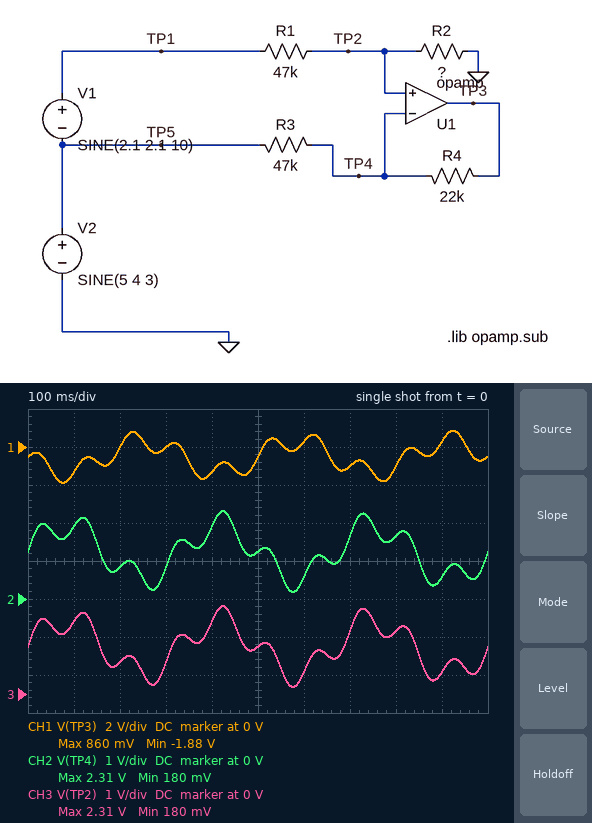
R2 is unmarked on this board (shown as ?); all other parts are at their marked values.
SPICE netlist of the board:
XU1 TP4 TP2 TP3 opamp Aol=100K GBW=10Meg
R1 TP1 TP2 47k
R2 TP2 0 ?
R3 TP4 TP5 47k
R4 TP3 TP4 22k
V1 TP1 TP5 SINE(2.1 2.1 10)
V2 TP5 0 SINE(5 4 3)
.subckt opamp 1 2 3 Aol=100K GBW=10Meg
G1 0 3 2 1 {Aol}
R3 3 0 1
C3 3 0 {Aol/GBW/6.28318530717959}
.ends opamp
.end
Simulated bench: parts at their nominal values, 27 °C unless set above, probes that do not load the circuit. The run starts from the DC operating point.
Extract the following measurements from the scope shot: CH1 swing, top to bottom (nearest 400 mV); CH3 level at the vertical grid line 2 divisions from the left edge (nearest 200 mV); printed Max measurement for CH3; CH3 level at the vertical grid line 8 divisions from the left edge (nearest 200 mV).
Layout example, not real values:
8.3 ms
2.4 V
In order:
2.8 V
800 mV
2.31 V
1.6 V
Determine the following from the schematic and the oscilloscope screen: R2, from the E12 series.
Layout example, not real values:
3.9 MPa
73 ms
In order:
10 kΩ
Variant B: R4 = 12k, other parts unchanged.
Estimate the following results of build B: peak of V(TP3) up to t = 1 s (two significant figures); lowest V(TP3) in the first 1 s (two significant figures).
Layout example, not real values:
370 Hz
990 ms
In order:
890 mV
-310 mV
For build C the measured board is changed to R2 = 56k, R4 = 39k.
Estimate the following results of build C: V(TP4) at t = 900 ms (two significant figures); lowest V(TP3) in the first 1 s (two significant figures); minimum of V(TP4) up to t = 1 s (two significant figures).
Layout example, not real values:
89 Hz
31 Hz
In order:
1.8 V
170 mV
570 mV
